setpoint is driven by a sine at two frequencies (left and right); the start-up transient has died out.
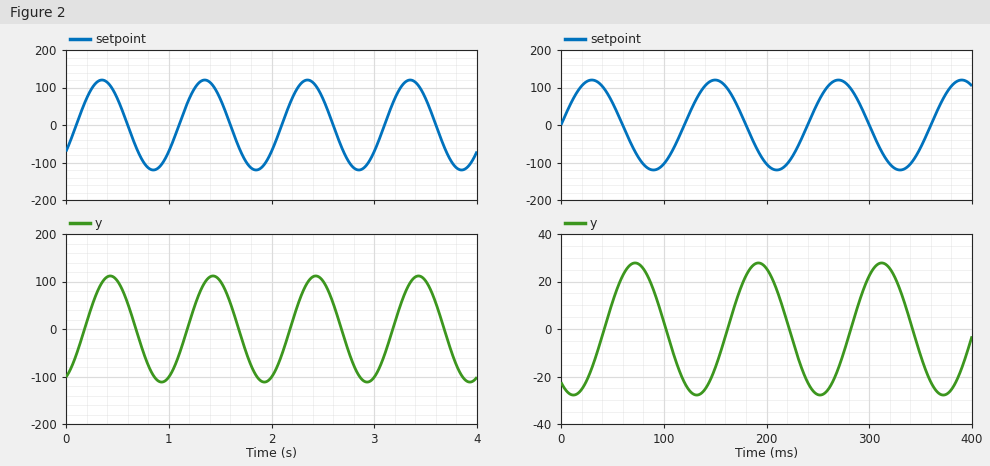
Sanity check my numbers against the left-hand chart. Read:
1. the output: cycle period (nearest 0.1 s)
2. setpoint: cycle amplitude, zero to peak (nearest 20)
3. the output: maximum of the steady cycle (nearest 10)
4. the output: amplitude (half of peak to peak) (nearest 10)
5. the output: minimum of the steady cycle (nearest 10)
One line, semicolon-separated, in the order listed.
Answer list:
1.0 s; 120; 110; 110; -110
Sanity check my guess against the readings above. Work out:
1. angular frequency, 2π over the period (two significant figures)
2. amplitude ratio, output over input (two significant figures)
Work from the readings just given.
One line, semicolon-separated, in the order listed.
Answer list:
6.3 rad/s; 0.92
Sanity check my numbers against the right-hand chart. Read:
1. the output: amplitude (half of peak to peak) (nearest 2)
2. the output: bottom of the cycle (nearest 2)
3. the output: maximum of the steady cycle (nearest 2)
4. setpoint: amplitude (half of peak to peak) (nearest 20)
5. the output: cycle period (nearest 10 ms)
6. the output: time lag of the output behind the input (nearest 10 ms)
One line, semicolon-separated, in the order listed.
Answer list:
28; -28; 28; 120; 120 ms; 40 ms
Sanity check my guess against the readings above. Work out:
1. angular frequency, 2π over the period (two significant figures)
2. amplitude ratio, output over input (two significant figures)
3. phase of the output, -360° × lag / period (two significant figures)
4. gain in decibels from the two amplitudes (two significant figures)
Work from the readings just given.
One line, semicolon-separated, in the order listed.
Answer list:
0.052 rad/ms; 0.23; -120°; -13 dB
